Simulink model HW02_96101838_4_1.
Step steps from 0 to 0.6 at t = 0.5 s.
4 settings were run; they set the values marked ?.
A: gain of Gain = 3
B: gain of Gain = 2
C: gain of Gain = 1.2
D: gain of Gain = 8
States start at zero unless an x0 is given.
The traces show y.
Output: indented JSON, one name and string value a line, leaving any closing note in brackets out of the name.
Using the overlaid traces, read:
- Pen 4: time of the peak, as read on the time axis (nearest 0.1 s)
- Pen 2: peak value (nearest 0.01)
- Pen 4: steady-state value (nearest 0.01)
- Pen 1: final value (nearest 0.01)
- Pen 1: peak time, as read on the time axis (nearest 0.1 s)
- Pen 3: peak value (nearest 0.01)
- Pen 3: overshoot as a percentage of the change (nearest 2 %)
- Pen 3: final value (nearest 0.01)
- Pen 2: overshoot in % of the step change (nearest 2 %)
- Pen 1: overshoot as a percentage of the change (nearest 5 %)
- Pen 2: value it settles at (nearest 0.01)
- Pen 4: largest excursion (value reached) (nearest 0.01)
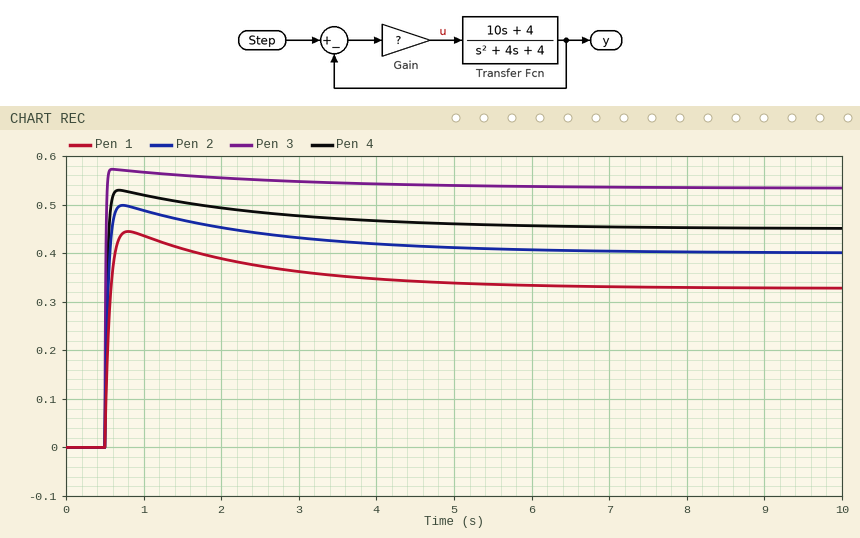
{
  "Pen 4: time of the peak, as read on the time axis": "0.7 s",
  "Pen 2: peak value": "0.50",
  "Pen 4: steady-state value": "0.45",
  "Pen 1: final value": "0.33",
  "Pen 1: peak time, as read on the time axis": "0.8 s",
  "Pen 3: peak value": "0.57",
  "Pen 3: overshoot as a percentage of the change": "8 %",
  "Pen 3: final value": "0.53",
  "Pen 2: overshoot in % of the step change": "24 %",
  "Pen 1: overshoot as a percentage of the change": "35 %",
  "Pen 2: value it settles at": "0.40",
  "Pen 4: largest excursion (value reached)": "0.53"
}
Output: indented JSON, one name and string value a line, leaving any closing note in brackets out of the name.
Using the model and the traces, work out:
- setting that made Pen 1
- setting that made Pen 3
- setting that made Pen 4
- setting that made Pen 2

{
  "setting that made Pen 1": "C",
  "setting that made Pen 3": "D",
  "setting that made Pen 4": "A",
  "setting that made Pen 2": "B"
}
